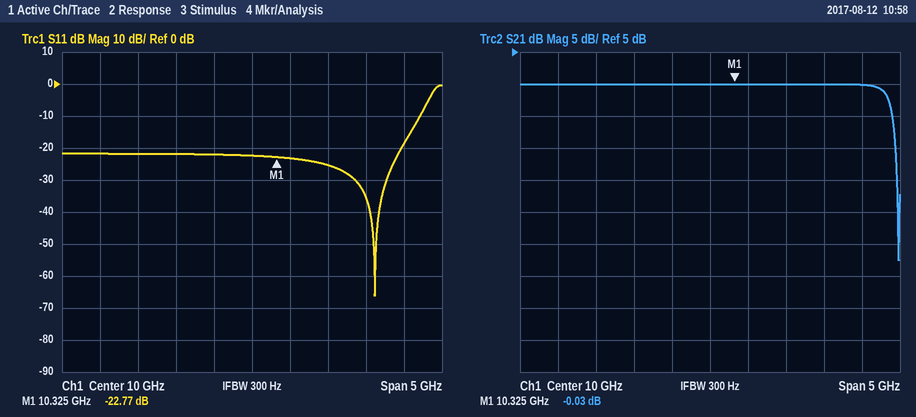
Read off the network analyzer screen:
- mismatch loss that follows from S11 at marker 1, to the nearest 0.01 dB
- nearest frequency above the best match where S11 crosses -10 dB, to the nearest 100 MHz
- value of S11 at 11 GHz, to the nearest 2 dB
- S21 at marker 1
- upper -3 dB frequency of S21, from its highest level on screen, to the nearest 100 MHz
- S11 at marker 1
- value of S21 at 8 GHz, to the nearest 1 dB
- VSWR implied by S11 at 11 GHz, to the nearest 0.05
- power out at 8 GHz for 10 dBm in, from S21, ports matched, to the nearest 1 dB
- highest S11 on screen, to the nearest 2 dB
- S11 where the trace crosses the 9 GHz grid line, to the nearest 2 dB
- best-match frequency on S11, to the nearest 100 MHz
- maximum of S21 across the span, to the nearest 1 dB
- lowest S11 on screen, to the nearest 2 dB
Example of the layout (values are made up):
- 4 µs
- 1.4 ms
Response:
- 0.02 dB
- 12.2 GHz
- -26 dB
- -0.03 dB
- 12.4 GHz
- -22.77 dB
- 0 dB
- 1.10
- 10 dBm
- 0 dB
- -22 dB
- 11.6 GHz
- 0 dB
- -66 dB
